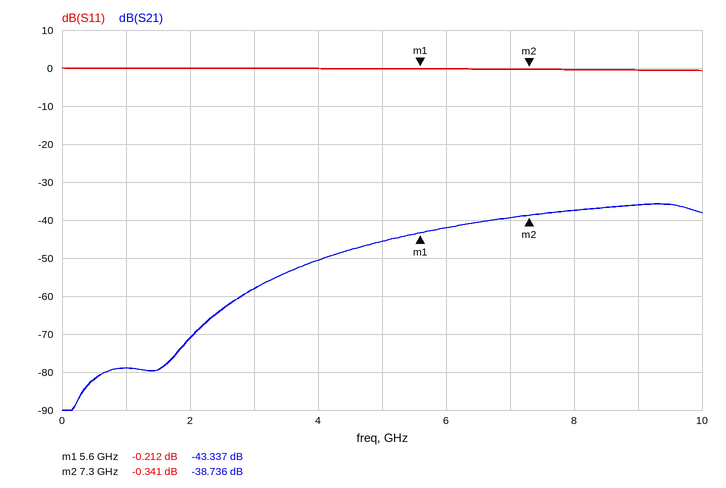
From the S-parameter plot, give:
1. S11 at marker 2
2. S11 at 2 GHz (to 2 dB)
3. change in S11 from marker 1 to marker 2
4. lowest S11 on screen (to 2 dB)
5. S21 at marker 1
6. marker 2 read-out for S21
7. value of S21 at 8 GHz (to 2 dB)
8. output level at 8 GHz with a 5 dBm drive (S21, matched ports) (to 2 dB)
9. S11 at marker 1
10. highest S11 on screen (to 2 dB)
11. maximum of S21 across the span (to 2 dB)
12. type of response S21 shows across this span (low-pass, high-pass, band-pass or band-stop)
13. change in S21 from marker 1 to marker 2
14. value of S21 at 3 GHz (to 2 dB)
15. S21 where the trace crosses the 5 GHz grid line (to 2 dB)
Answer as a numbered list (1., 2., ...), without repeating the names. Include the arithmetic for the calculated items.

1. -0.341 dB
2. 0 dB
3. -0.341 − (-0.212) = -0.129 dB
4. 0 dB
5. -43.337 dB
6. -38.736 dB
7. -38 dB
8. 5 dBm + (-38 dB) = -32 dBm
9. -0.212 dB
10. 0 dB
11. -36 dB
12. high-pass
13. -38.736 − (-43.337) = 4.601 dB
14. -58 dB
15. -46 dB
